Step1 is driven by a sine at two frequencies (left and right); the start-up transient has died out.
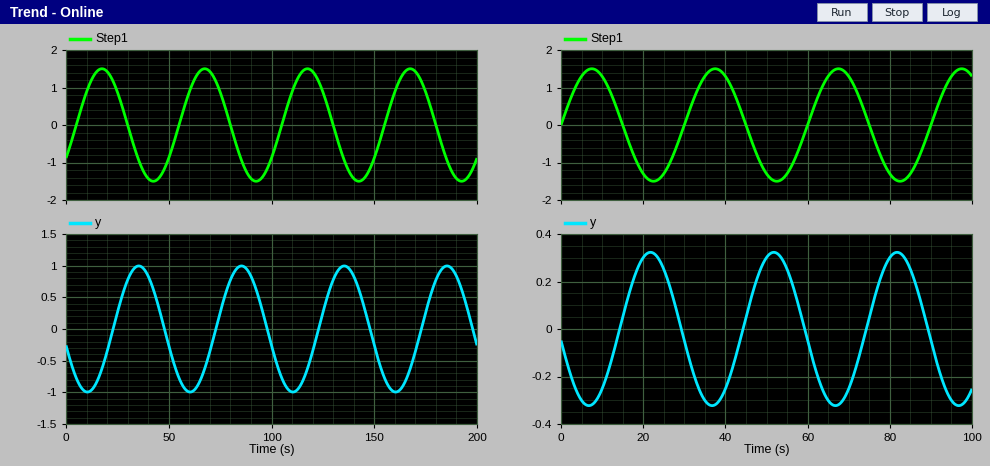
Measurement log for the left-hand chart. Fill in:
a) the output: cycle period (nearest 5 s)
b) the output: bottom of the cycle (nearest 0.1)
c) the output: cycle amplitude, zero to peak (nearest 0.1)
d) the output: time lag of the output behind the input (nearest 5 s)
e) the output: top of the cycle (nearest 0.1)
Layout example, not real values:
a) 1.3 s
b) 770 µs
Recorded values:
a) 50 s
b) -1.0
c) 1.0
d) 20 s
e) 1.0
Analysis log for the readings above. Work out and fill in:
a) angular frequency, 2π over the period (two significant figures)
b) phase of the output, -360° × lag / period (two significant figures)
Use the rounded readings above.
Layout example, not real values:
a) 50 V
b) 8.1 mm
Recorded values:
a) 0.13 rad/s
b) -140°
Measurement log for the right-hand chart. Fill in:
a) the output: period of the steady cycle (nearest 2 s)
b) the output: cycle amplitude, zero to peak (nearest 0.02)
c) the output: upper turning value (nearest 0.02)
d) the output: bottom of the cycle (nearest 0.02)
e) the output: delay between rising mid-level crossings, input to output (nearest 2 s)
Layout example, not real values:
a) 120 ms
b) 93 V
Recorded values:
a) 30 s
b) 0.32
c) 0.32
d) -0.32
e) 14 s
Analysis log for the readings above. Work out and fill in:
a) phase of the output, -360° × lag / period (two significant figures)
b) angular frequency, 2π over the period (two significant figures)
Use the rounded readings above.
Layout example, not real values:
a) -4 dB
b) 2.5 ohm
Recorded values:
a) -170°
b) 0.21 rad/s
